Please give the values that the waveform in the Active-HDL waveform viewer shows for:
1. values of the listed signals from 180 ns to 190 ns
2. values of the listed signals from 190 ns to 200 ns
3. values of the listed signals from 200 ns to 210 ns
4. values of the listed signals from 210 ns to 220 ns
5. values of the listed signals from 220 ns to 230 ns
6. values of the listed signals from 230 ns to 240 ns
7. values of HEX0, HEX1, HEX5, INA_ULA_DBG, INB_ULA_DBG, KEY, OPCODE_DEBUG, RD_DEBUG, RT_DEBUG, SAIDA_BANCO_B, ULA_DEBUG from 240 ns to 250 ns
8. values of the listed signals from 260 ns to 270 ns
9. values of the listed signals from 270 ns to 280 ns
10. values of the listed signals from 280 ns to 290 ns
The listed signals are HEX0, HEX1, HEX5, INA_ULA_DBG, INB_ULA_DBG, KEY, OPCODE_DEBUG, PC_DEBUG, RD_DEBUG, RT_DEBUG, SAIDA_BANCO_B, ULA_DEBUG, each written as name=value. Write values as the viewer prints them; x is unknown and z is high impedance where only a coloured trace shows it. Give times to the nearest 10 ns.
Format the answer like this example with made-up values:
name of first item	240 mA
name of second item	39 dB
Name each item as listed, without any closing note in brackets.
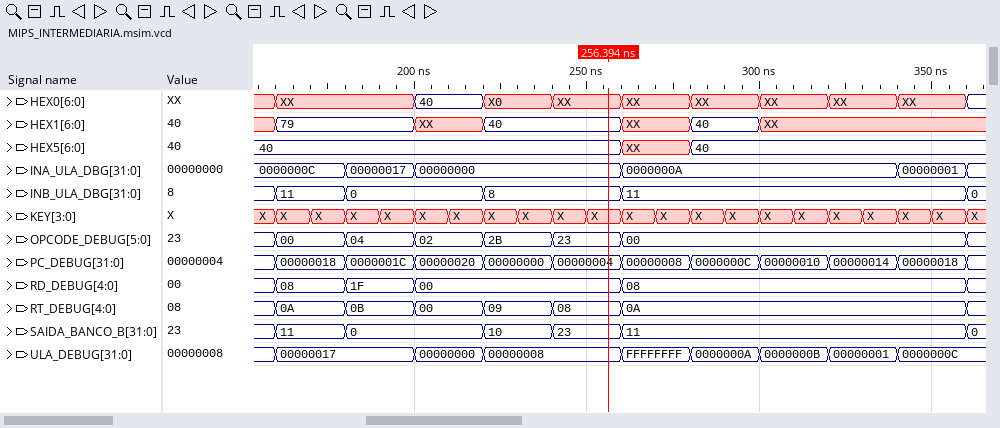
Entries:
values of the listed signals from 180 ns to 190 ns	HEX0=XX, HEX1=79, HEX5=40, INA_ULA_DBG=00000017, INB_ULA_DBG=0, KEY=X, OPCODE_DEBUG=04, PC_DEBUG=0000001C, RD_DEBUG=1F, RT_DEBUG=0B, SAIDA_BANCO_B=0, ULA_DEBUG=00000017
values of the listed signals from 190 ns to 200 ns	HEX0=XX, HEX1=79, HEX5=40, INA_ULA_DBG=00000017, INB_ULA_DBG=0, KEY=X, OPCODE_DEBUG=04, PC_DEBUG=0000001C, RD_DEBUG=1F, RT_DEBUG=0B, SAIDA_BANCO_B=0, ULA_DEBUG=00000017
values of the listed signals from 200 ns to 210 ns	HEX0=40, HEX1=XX, HEX5=40, INA_ULA_DBG=00000000, INB_ULA_DBG=0, KEY=X, OPCODE_DEBUG=02, PC_DEBUG=00000020, RD_DEBUG=00, RT_DEBUG=00, SAIDA_BANCO_B=0, ULA_DEBUG=00000000
values of the listed signals from 210 ns to 220 ns	HEX0=40, HEX1=XX, HEX5=40, INA_ULA_DBG=00000000, INB_ULA_DBG=0, KEY=X, OPCODE_DEBUG=02, PC_DEBUG=00000020, RD_DEBUG=00, RT_DEBUG=00, SAIDA_BANCO_B=0, ULA_DEBUG=00000000
values of the listed signals from 220 ns to 230 ns	HEX0=X0, HEX1=40, HEX5=40, INA_ULA_DBG=00000000, INB_ULA_DBG=8, KEY=X, OPCODE_DEBUG=2B, PC_DEBUG=00000000, RD_DEBUG=00, RT_DEBUG=09, SAIDA_BANCO_B=10, ULA_DEBUG=00000008
values of the listed signals from 230 ns to 240 ns	HEX0=X0, HEX1=40, HEX5=40, INA_ULA_DBG=00000000, INB_ULA_DBG=8, KEY=X, OPCODE_DEBUG=2B, PC_DEBUG=00000000, RD_DEBUG=00, RT_DEBUG=09, SAIDA_BANCO_B=10, ULA_DEBUG=00000008
values of HEX0, HEX1, HEX5, INA_ULA_DBG, INB_ULA_DBG, KEY, OPCODE_DEBUG, RD_DEBUG, RT_DEBUG, SAIDA_BANCO_B, ULA_DEBUG from 240 ns to 250 ns	HEX0=XX, HEX1=40, HEX5=40, INA_ULA_DBG=00000000, INB_ULA_DBG=8, KEY=X, OPCODE_DEBUG=23, RD_DEBUG=00, RT_DEBUG=08, SAIDA_BANCO_B=23, ULA_DEBUG=00000008
values of the listed signals from 260 ns to 270 ns	HEX0=XX, HEX1=XX, HEX5=XX, INA_ULA_DBG=0000000A, INB_ULA_DBG=11, KEY=X, OPCODE_DEBUG=00, PC_DEBUG=00000008, RD_DEBUG=08, RT_DEBUG=0A, SAIDA_BANCO_B=11, ULA_DEBUG=FFFFFFFF
values of the listed signals from 270 ns to 280 ns	HEX0=XX, HEX1=XX, HEX5=XX, INA_ULA_DBG=0000000A, INB_ULA_DBG=11, KEY=X, OPCODE_DEBUG=00, PC_DEBUG=00000008, RD_DEBUG=08, RT_DEBUG=0A, SAIDA_BANCO_B=11, ULA_DEBUG=FFFFFFFF
values of the listed signals from 280 ns to 290 ns	HEX0=XX, HEX1=40, HEX5=40, INA_ULA_DBG=0000000A, INB_ULA_DBG=11, KEY=X, OPCODE_DEBUG=00, PC_DEBUG=0000000C, RD_DEBUG=08, RT_DEBUG=0A, SAIDA_BANCO_B=11, ULA_DEBUG=0000000A
